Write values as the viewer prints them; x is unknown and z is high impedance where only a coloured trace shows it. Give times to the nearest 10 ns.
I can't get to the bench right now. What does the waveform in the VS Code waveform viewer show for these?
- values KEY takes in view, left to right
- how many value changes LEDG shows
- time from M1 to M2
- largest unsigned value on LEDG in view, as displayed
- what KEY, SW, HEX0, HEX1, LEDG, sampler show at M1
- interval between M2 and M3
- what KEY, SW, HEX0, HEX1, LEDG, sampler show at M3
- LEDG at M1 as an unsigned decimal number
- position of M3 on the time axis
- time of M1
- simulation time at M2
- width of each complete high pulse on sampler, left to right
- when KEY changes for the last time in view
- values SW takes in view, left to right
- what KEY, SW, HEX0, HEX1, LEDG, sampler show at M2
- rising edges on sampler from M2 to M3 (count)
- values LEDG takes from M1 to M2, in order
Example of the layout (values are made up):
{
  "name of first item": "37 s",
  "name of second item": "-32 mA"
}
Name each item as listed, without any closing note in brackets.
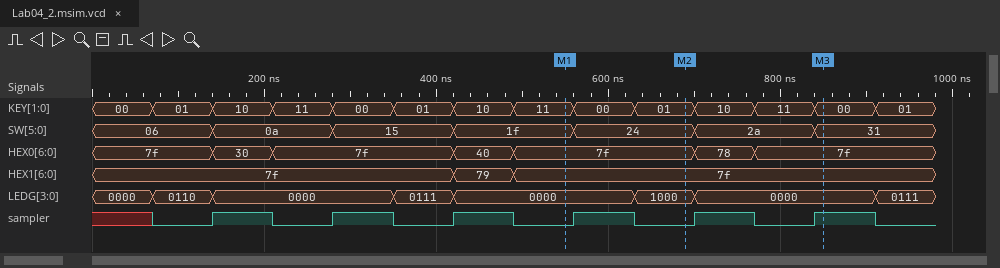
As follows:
{
  "values KEY takes in view, left to right": "00, 01, 10, 11, 00, 01, 10, 11, 00, 01, 10, 11, 00, 01",
  "how many value changes LEDG shows": "7",
  "time from M1 to M2": "140 ns",
  "largest unsigned value on LEDG in view, as displayed": "1000",
  "what KEY, SW, HEX0, HEX1, LEDG, sampler show at M1": "KEY=11, SW=1f, HEX0=7f, HEX1=7f, LEDG=0000, sampler=0",
  "interval between M2 and M3": "160 ns",
  "what KEY, SW, HEX0, HEX1, LEDG, sampler show at M3": "KEY=00, SW=31, HEX0=7f, HEX1=7f, LEDG=0000, sampler=1",
  "LEDG at M1 as an unsigned decimal number": "0",
  "position of M3 on the time axis": "850 ns",
  "time of M1": "550 ns",
  "simulation time at M2": "690 ns",
  "width of each complete high pulse on sampler, left to right": "70 ns, 70 ns, 70 ns, 70 ns, 70 ns, 70 ns",
  "when KEY changes for the last time in view": "910 ns",
  "values SW takes in view, left to right": "06, 0a, 15, 1f, 24, 2a, 31",
  "what KEY, SW, HEX0, HEX1, LEDG, sampler show at M2": "KEY=01, SW=24, HEX0=7f, HEX1=7f, LEDG=1000, sampler=0",
  "rising edges on sampler from M2 to M3": "2",
  "values LEDG takes from M1 to M2, in order": "0000, 1000"
}
